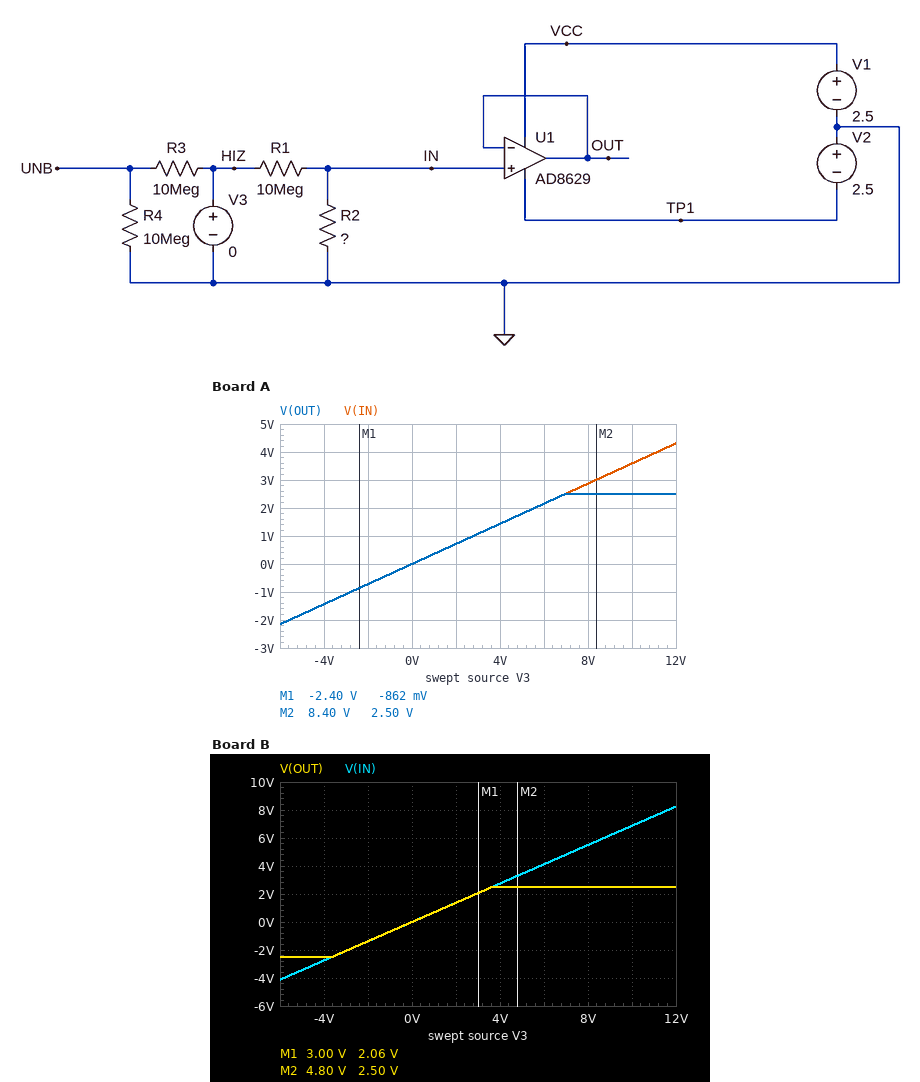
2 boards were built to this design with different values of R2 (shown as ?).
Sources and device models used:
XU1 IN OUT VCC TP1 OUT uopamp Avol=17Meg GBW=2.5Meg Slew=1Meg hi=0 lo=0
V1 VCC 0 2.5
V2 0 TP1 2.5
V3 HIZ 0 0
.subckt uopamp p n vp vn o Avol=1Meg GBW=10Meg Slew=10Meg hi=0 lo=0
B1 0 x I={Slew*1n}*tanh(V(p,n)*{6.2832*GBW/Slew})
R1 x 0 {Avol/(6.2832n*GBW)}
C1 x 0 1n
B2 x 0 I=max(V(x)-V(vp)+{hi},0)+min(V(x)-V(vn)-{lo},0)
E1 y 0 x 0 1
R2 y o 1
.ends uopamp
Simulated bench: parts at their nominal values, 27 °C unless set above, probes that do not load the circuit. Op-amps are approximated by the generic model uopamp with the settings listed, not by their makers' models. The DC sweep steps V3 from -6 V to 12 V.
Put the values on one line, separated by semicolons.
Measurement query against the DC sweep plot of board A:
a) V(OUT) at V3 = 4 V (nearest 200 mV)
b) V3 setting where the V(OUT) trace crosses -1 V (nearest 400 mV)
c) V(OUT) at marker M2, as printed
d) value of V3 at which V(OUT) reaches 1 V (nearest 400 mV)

1.4 V; -2.8 V; 2.50 V; 2.8 V
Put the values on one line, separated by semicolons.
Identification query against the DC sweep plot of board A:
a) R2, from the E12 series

5.6 MΩ
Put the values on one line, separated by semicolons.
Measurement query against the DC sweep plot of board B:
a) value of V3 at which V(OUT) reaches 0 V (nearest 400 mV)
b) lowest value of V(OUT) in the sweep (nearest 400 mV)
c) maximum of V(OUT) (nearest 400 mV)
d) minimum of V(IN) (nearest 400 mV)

0 V; -2.4 V; 2.4 V; -4.0 V
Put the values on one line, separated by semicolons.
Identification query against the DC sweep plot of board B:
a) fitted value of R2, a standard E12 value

22 MΩ
